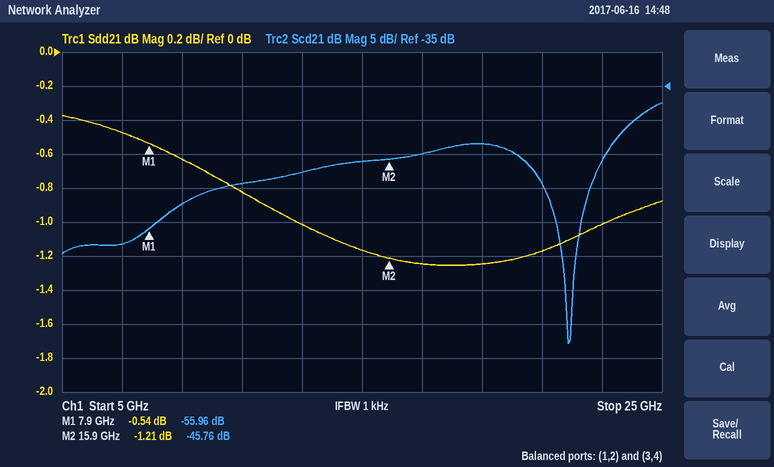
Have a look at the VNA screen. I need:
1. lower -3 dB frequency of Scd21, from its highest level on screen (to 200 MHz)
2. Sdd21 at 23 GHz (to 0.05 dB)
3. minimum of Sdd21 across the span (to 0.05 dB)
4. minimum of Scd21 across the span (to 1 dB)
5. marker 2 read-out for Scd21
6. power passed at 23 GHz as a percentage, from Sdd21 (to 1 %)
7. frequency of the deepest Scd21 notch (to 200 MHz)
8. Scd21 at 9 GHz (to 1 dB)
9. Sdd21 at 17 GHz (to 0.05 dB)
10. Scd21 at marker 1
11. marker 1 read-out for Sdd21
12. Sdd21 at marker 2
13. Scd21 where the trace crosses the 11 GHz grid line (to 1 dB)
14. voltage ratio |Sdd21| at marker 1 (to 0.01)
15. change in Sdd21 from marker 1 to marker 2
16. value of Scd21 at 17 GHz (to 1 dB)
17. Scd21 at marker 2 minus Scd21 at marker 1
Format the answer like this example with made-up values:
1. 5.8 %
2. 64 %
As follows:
1. 24.0 GHz
2. -1.00 dB
3. -1.25 dB
4. -73 dB
5. -45.76 dB
6. 79 %
7. 21.8 GHz
8. -52 dB
9. -1.25 dB
10. -55.96 dB
11. -0.54 dB
12. -1.21 dB
13. -49 dB
14. 0.94
15. -0.67 dB
16. -45 dB
17. 10.20 dB
